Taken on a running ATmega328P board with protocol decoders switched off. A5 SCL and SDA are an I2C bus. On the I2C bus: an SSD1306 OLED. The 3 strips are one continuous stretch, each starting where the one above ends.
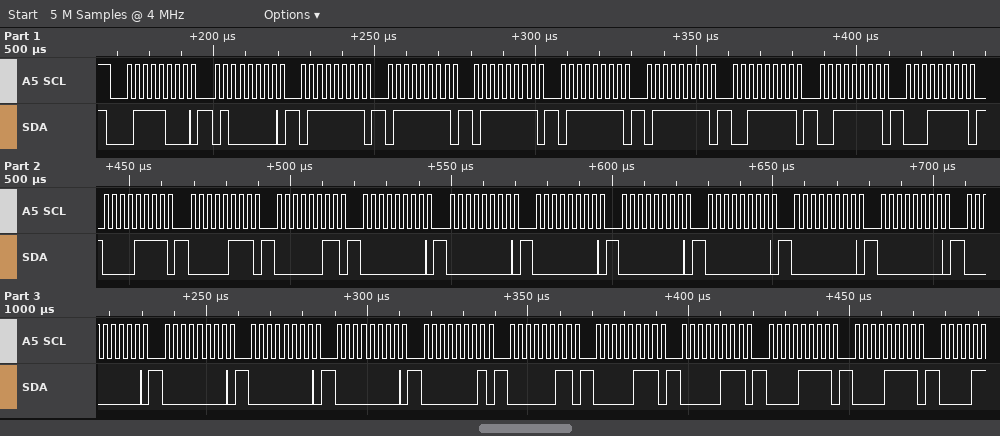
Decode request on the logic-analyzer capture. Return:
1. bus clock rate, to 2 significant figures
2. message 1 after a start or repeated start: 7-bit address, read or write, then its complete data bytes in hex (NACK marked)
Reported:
400 kHz
0x3C write: 40 7F 7F 7F 7F 7F 3F 3F 1F 0F 07 03 00 00 00 00 00 00 00 00 00 00 00 01 03 07 07 0F 0F
